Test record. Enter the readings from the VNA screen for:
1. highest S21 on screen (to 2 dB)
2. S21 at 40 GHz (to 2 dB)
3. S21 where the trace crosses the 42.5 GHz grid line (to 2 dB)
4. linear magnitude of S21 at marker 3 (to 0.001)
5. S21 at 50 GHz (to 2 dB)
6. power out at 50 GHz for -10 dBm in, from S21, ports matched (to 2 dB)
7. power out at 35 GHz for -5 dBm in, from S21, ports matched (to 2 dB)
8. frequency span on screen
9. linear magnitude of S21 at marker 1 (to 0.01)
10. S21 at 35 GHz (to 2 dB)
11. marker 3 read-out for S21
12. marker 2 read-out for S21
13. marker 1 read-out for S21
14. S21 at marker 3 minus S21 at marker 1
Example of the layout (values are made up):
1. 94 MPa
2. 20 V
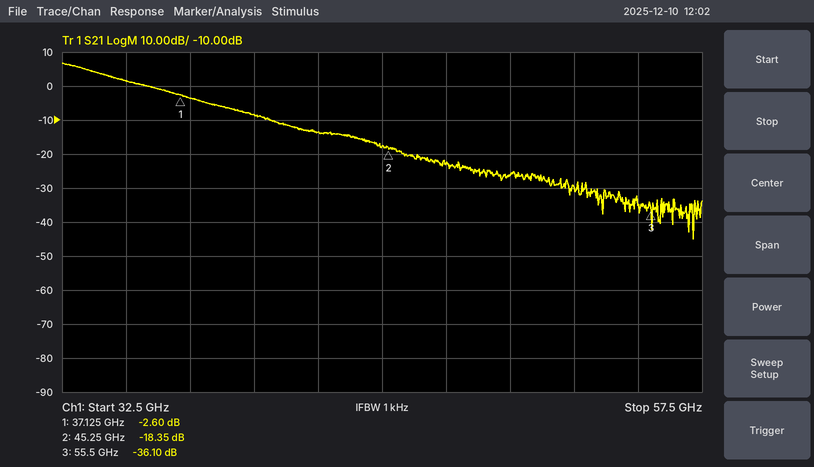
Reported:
1. 6 dB
2. -8 dB
3. -14 dB
4. 0.016
5. -26 dB
6. -36 dBm
7. -4 dBm
8. 25 GHz
9. 0.74
10. 2 dB
11. -36.10 dB
12. -18.35 dB
13. -2.60 dB
14. -33.50 dB
